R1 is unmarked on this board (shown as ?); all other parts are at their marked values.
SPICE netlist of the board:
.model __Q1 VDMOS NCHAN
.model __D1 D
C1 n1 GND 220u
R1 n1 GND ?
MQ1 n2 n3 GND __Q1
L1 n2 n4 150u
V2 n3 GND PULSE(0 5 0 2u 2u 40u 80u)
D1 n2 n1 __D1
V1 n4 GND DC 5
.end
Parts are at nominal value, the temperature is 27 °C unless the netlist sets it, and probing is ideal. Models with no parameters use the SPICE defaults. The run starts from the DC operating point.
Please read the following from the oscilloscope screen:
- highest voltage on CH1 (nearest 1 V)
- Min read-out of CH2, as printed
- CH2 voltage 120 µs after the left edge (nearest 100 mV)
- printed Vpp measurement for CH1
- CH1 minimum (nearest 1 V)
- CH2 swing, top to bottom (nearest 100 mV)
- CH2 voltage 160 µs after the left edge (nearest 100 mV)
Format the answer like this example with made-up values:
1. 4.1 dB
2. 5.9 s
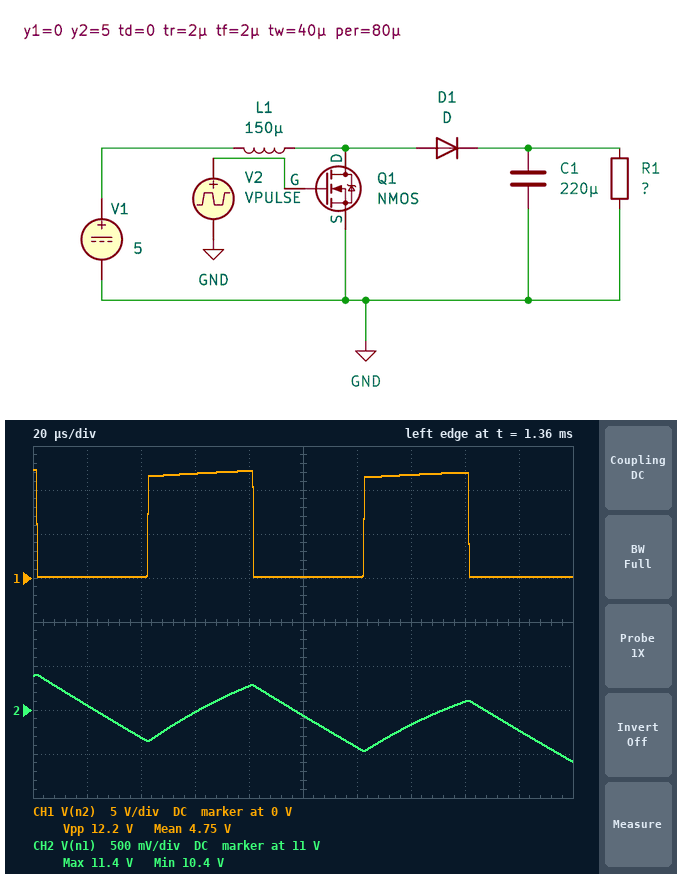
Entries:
1. 12 V
2. 10.4 V
3. 10.6 V
4. 12.2 V
5. 0 V
6. 1.0 V
7. 11.1 V
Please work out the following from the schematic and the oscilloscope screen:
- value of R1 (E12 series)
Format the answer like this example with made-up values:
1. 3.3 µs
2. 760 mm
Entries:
1. 2.7 Ω
